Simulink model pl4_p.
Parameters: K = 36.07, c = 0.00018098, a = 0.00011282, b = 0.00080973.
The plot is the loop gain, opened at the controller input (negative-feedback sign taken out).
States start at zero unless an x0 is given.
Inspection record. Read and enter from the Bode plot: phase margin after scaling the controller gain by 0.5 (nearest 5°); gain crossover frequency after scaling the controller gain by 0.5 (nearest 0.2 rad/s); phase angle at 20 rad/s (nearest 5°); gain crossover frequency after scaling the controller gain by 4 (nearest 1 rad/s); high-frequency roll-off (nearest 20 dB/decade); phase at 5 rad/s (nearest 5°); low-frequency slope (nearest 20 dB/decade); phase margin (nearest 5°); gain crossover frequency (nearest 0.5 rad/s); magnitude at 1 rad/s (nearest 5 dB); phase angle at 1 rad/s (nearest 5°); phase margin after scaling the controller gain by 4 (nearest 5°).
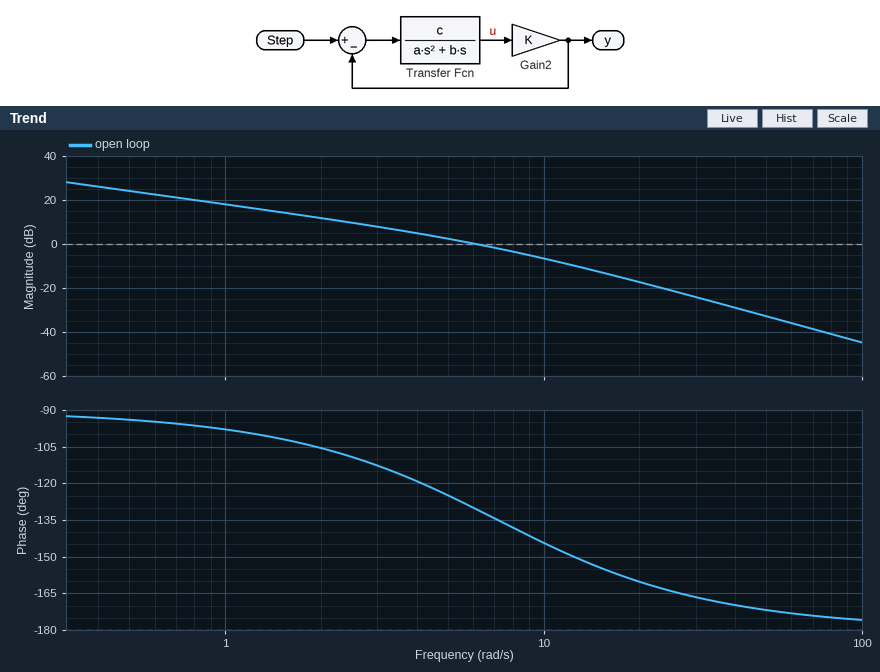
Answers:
65°
3.6 rad/s
-160°
14 rad/s
-40 dB/decade
-125°
-20 dB/decade
50°
6.0 rad/s
20 dB
-100°
25°
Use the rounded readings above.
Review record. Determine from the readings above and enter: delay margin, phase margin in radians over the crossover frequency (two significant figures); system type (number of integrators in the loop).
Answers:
0.15 s
1
